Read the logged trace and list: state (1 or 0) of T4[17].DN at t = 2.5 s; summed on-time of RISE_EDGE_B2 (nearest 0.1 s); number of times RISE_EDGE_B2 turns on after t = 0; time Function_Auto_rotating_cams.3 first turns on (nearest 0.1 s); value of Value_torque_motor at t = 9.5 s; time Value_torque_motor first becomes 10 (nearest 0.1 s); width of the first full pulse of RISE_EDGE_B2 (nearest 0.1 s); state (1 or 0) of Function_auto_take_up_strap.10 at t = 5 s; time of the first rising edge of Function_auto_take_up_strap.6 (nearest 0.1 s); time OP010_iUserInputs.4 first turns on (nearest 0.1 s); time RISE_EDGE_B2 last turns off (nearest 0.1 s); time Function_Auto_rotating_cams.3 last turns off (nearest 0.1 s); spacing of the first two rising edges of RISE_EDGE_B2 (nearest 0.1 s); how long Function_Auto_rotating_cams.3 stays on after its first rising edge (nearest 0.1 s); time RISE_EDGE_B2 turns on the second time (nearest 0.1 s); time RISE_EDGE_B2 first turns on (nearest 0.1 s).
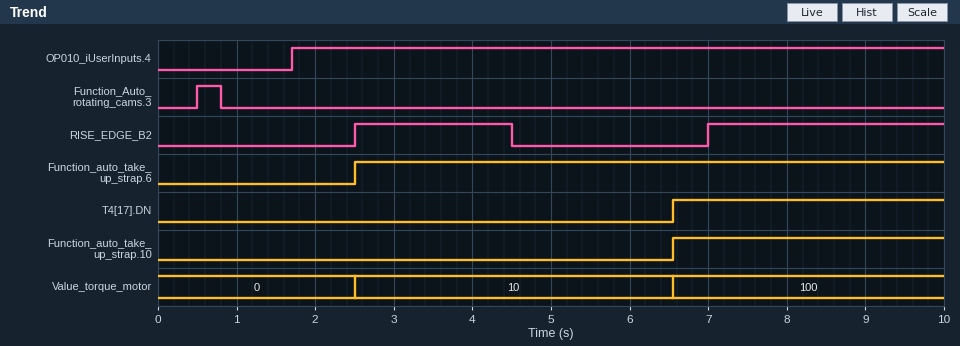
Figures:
0
5.0 s
2
0.5 s
100
2.5 s
2.0 s
0
2.5 s
1.7 s
4.5 s
0.8 s
4.5 s
0.3 s
7.0 s
2.5 s
